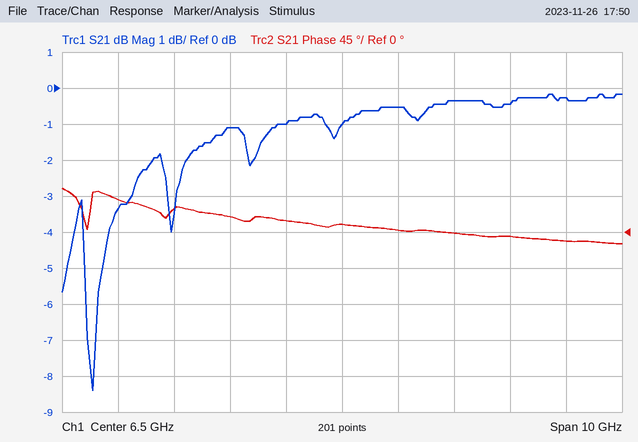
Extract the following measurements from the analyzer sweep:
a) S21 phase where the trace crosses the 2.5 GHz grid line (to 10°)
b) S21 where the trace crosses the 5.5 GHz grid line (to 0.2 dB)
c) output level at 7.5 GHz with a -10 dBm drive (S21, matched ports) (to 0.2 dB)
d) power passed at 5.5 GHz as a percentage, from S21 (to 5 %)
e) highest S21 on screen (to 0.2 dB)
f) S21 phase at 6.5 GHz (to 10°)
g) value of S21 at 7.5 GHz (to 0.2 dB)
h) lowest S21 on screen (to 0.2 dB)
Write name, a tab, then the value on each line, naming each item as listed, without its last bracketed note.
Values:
S21 phase where the trace crosses the 2.5 GHz grid line	40°
S21 where the trace crosses the 5.5 GHz grid line	-1.0 dB
output level at 7.5 GHz with a -10 dBm drive (S21, matched ports)	-10.6 dBm
power passed at 5.5 GHz as a percentage, from S21	80 %
highest S21 on screen	-0.2 dB
S21 phase at 6.5 GHz	10°
value of S21 at 7.5 GHz	-0.6 dB
lowest S21 on screen	-8.4 dB
